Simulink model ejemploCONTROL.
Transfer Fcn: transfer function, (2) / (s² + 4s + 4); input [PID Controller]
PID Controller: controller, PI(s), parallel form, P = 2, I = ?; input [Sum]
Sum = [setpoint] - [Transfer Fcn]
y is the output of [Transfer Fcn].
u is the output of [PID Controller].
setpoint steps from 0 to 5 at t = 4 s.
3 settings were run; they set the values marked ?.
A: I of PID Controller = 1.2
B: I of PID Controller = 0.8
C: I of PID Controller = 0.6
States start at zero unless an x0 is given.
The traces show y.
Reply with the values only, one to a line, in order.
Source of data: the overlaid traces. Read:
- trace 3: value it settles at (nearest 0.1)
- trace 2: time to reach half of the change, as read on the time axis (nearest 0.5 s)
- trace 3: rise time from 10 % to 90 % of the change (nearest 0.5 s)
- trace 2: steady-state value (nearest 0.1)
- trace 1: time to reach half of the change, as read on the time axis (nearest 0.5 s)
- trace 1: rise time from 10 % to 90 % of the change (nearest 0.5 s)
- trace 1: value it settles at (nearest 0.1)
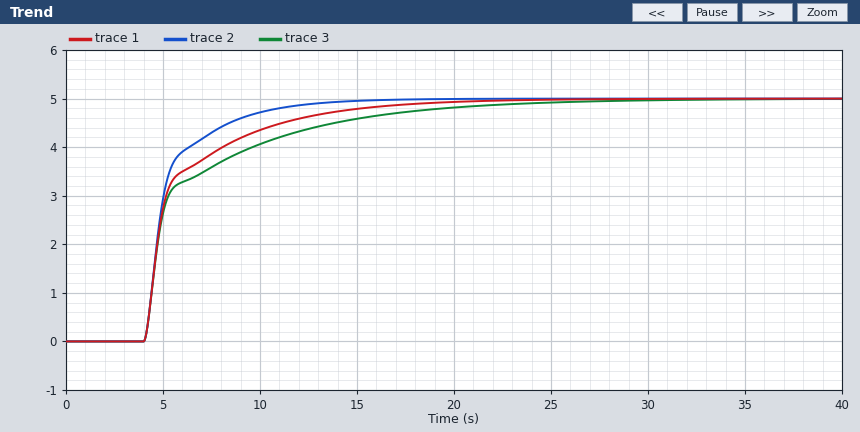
5.0
5.0 s
9.5 s
5.0
5.0 s
7.0 s
5.0
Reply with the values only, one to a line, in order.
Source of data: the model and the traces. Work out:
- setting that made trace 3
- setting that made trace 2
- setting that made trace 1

C
A
B
